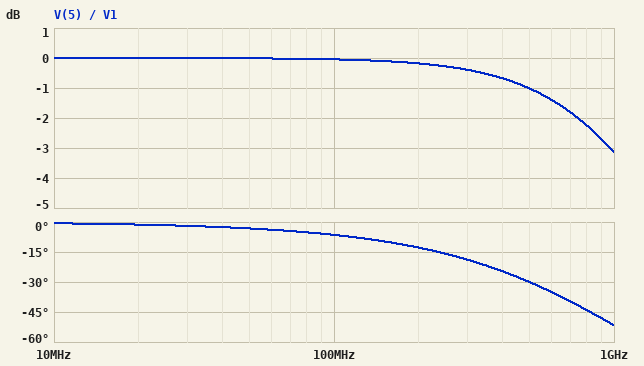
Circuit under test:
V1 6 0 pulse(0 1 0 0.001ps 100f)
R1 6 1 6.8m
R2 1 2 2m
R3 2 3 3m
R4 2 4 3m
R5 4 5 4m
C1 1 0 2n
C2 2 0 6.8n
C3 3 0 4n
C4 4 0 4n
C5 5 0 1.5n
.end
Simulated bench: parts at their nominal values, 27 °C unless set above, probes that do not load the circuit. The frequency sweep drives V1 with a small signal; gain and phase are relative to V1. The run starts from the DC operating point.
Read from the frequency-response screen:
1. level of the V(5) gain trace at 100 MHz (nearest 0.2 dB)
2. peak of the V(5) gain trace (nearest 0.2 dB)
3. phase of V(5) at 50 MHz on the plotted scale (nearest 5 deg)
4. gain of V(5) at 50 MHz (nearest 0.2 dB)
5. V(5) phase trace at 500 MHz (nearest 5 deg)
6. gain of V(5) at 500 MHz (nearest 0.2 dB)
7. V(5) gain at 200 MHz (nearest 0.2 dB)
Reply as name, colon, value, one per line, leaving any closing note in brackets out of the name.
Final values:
level of the V(5) gain trace at 100 MHz: 0 dB
peak of the V(5) gain trace: 0 dB
phase of V(5) at 50 MHz on the plotted scale: -5 deg
gain of V(5) at 50 MHz: 0 dB
V(5) phase trace at 500 MHz: -30 deg
gain of V(5) at 500 MHz: -1.0 dB
V(5) gain at 200 MHz: -0.2 dB
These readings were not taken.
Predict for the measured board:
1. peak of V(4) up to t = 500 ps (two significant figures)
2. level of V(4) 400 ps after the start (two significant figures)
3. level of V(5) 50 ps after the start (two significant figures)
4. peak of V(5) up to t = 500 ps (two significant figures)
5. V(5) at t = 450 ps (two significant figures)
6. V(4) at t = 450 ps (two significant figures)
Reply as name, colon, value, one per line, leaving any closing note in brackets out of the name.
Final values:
peak of V(4) up to t = 500 ps: 950 mV
level of V(4) 400 ps after the start: 910 mV
level of V(5) 50 ps after the start: 190 mV
peak of V(5) up to t = 500 ps: 950 mV
V(5) at t = 450 ps: 930 mV
V(4) at t = 450 ps: 930 mV
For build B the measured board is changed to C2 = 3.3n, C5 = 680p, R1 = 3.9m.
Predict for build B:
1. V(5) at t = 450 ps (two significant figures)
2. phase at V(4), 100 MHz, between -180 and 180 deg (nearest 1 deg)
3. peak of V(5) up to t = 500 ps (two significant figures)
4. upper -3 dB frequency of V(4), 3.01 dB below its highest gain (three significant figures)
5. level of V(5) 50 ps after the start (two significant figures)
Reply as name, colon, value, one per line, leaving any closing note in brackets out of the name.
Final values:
V(5) at t = 450 ps: 990 mV
phase at V(4), 100 MHz, between -180 and 180 deg: -3 deg
peak of V(5) up to t = 500 ps: 1.0 V
upper -3 dB frequency of V(4), 3.01 dB below its highest gain: 1.85 GHz
level of V(5) 50 ps after the start: 370 mV
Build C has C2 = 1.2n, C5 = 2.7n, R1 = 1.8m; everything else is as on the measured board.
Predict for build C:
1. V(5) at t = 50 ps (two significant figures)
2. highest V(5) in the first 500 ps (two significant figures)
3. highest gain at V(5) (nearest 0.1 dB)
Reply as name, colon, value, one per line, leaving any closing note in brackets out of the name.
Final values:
V(5) at t = 50 ps: 420 mV
highest V(5) in the first 500 ps: 1.0 V
highest gain at V(5): 0 dB
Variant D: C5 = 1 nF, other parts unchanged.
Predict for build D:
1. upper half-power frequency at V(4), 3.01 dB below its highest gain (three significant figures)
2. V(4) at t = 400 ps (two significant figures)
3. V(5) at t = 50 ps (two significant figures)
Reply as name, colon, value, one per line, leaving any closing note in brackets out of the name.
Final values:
upper half-power frequency at V(4), 3.01 dB below its highest gain: 1.01 GHz
V(4) at t = 400 ps: 920 mV
V(5) at t = 50 ps: 200 mV
